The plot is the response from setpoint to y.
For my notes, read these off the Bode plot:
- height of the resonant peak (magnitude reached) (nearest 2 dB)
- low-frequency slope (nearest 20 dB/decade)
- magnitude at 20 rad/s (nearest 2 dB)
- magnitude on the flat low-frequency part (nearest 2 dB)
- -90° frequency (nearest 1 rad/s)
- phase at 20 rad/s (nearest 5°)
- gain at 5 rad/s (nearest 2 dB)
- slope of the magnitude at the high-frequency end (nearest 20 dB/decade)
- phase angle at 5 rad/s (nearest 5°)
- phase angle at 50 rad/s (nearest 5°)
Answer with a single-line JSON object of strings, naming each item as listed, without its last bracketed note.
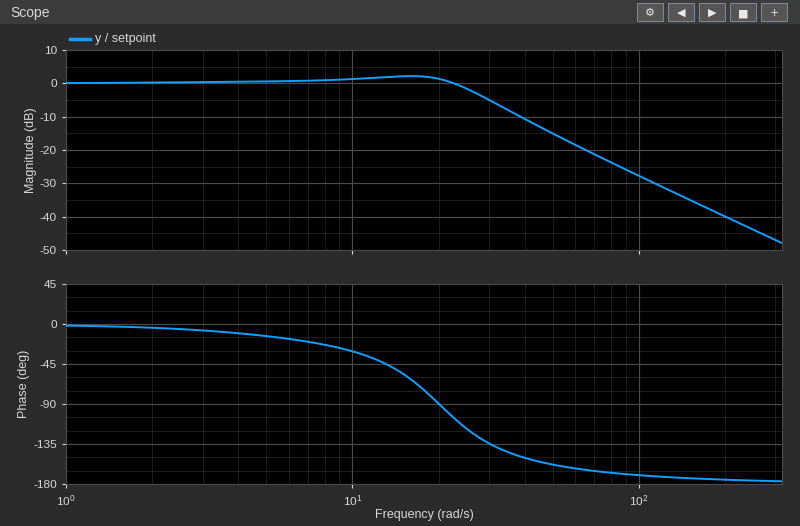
{"height of the resonant peak (magnitude reached)": "2 dB", "low-frequency slope": "0 dB/decade", "magnitude at 20 rad/s": "2 dB", "magnitude on the flat low-frequency part": "0 dB", "-90° frequency": "20 rad/s", "phase at 20 rad/s": "-90°", "gain at 5 rad/s": "0 dB", "slope of the magnitude at the high-frequency end": "-40 dB/decade", "phase angle at 5 rad/s": "-15°", "phase angle at 50 rad/s": "-160°"}
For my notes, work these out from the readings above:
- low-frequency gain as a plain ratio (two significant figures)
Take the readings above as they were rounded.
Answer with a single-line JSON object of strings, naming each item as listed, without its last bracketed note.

{"low-frequency gain as a plain ratio": "1.0"}
